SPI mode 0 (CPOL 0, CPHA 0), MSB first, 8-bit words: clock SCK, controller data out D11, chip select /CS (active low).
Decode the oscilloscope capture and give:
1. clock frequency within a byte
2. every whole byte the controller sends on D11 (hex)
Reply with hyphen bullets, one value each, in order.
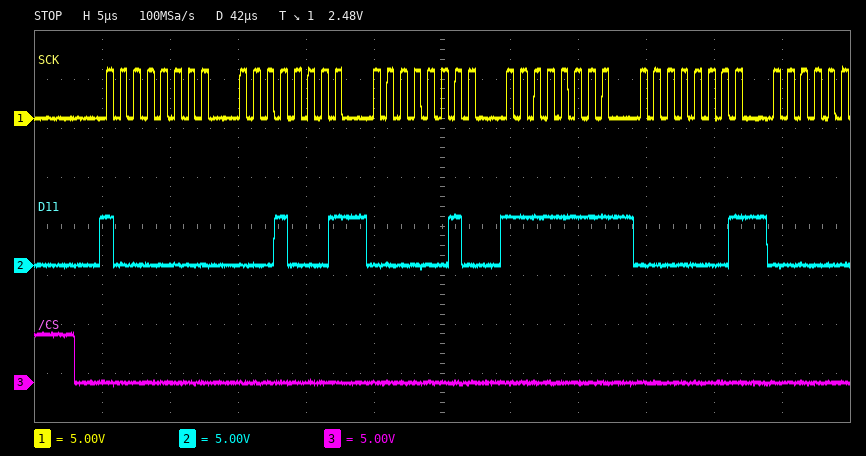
- 1 MHz
- 0x80 0x11 0x02 0xFF 0x01
